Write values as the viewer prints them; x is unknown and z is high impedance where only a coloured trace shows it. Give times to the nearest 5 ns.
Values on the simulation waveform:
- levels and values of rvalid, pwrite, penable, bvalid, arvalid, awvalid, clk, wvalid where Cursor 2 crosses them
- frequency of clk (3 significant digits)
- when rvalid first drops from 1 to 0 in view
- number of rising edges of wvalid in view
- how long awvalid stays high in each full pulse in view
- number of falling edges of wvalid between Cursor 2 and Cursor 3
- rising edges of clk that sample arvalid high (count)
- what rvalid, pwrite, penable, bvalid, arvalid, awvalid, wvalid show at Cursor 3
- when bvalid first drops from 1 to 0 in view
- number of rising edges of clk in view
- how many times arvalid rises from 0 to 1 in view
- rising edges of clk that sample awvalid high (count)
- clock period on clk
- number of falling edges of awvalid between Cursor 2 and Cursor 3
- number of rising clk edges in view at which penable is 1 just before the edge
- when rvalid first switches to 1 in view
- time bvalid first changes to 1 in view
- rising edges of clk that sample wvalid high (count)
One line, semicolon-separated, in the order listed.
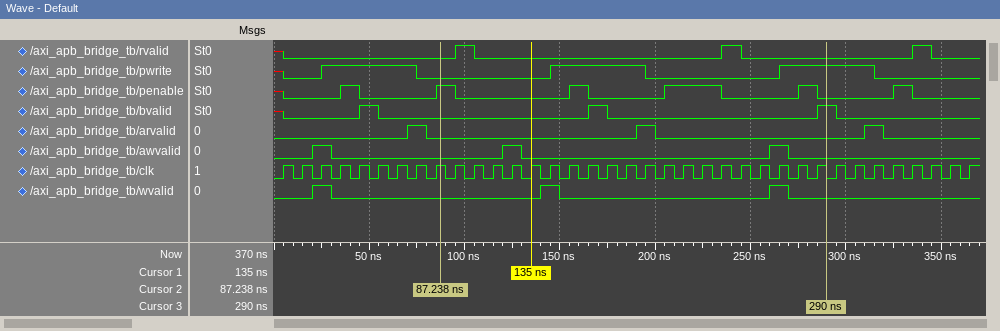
rvalid=0, pwrite=0, penable=1, bvalid=0, arvalid=0, awvalid=0, clk=1, wvalid=0; 100 MHz; 105 ns; 3; 10 ns, 10 ns, 10 ns; 2; 3; rvalid=0, pwrite=1, penable=0, bvalid=1, arvalid=0, awvalid=0, wvalid=0; 55 ns; 37; 3; 3; 10 ns; 2; 8; 95 ns; 45 ns; 3
